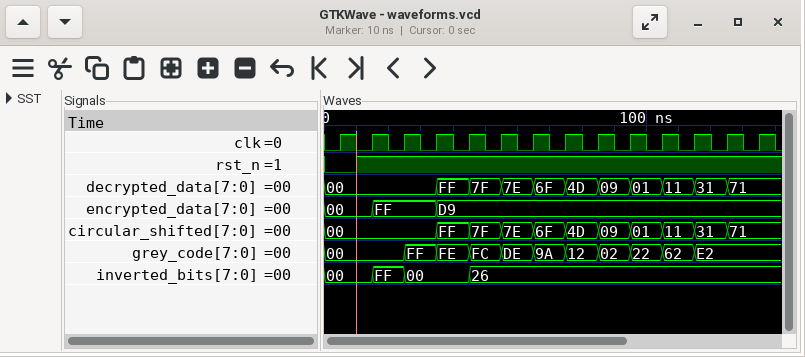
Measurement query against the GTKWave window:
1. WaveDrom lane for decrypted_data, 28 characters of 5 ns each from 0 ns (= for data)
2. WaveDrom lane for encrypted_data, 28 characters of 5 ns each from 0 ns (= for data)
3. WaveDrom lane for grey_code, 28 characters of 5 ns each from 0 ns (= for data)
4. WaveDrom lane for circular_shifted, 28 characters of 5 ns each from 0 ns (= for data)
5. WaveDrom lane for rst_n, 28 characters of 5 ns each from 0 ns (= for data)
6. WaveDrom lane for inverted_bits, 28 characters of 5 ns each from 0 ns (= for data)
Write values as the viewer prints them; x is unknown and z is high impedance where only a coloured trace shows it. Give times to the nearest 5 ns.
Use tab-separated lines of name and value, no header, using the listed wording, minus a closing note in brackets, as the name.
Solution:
WaveDrom lane for decrypted_data, 28 characters of 5 ns each from 0 ns	{name: 'decrypted_data', wave: '=......=.=.=.=.=.=.=.=.=.=..', data: '00 FF 7F 7E 6F 4D 09 01 11 31 71'}
WaveDrom lane for encrypted_data, 28 characters of 5 ns each from 0 ns	{name: 'encrypted_data', wave: '=..=...=....................', data: '00 FF D9'}
WaveDrom lane for grey_code, 28 characters of 5 ns each from 0 ns	{name: 'grey_code', wave: '=....=.=.=.=.=.=.=.=.=.=....', data: '00 FF FE FC DE 9A 12 02 22 62 E2'}
WaveDrom lane for circular_shifted, 28 characters of 5 ns each from 0 ns	{name: 'circular_shifted', wave: '=......=.=.=.=.=.=.=.=.=.=..', data: '00 FF 7F 7E 6F 4D 09 01 11 31 71'}
WaveDrom lane for rst_n, 28 characters of 5 ns each from 0 ns	{name: 'rst_n', wave: '0.1.........................'}
WaveDrom lane for inverted_bits, 28 characters of 5 ns each from 0 ns	{name: 'inverted_bits', wave: '=..=.=...=..................', data: '00 FF 00 26'}
